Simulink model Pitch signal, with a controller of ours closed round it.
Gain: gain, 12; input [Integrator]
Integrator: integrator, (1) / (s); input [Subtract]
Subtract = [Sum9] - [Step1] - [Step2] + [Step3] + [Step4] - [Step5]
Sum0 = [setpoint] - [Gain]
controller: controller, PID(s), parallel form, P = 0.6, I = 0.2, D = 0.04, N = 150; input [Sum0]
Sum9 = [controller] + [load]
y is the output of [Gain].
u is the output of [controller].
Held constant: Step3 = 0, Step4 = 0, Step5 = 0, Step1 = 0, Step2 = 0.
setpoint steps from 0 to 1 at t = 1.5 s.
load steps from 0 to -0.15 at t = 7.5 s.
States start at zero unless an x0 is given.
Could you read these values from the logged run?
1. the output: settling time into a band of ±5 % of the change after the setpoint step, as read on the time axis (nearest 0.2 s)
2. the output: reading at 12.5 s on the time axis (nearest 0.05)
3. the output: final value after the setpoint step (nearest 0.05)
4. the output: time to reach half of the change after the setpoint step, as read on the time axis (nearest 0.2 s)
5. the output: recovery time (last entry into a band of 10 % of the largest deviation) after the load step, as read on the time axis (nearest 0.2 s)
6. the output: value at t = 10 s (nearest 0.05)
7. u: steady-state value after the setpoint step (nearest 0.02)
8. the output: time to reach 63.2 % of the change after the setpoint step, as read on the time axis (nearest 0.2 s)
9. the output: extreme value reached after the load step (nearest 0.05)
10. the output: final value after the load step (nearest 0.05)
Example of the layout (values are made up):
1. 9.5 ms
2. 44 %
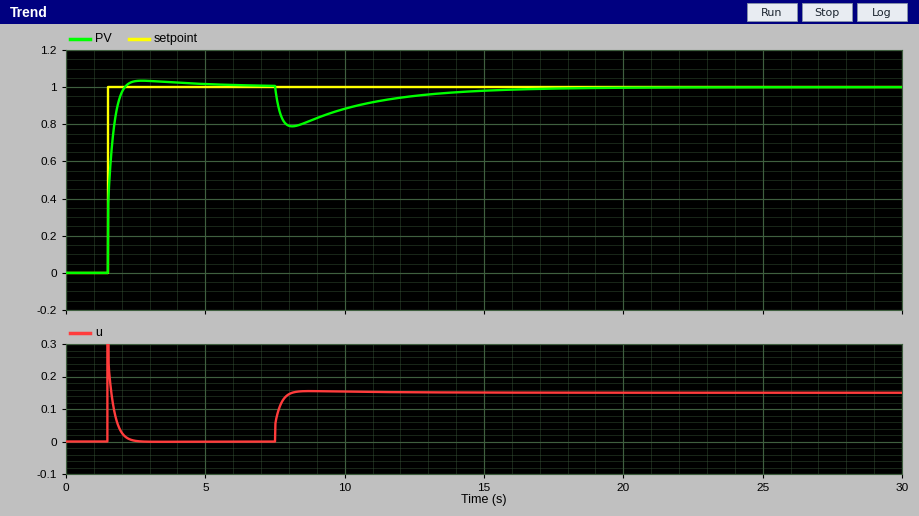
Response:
1. 2.0 s
2. 0.95
3. 1.00
4. 1.6 s
5. 14.6 s
6. 0.90
7. 0.00
8. 1.6 s
9. 0.80
10. 1.00
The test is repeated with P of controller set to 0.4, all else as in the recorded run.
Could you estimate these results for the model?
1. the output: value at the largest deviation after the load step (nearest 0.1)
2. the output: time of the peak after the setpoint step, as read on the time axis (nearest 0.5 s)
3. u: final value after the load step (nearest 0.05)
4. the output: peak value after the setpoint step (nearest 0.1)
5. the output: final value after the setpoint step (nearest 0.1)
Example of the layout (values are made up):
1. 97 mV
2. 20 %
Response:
1. 0.7
2. 3.0 s
3. 0.15
4. 1.1
5. 1.0
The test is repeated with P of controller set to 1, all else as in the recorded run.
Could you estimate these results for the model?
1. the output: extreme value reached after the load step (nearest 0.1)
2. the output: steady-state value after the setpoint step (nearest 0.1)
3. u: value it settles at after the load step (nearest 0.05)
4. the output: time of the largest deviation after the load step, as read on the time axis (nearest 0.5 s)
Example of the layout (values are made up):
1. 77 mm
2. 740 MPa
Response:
1. 0.9
2. 1.0
3. 0.15
4. 8.0 s
